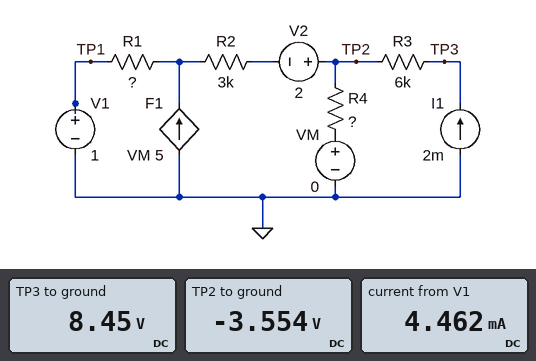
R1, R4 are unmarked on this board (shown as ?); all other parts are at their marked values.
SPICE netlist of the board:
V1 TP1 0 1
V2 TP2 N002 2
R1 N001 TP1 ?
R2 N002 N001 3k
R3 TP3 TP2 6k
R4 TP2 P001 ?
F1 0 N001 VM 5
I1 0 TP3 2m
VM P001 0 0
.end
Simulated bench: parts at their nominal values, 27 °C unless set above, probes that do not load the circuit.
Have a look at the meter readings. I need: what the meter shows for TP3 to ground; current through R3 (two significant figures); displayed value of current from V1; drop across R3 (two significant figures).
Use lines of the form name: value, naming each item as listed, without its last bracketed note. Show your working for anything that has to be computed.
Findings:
what the meter shows for TP3 to ground: 8.45 V
current through R3: (8.45 V - (-3.554 V)) / 6 kΩ = 2.0 mA
displayed value of current from V1: 4.462 mA
drop across R3: 8.45 V - (-3.554 V) = 12 V
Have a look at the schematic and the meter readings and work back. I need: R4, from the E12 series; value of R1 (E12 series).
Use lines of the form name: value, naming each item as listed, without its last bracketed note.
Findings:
R4, from the E12 series: 2.2 kΩ
value of R1: 3.9 kΩ
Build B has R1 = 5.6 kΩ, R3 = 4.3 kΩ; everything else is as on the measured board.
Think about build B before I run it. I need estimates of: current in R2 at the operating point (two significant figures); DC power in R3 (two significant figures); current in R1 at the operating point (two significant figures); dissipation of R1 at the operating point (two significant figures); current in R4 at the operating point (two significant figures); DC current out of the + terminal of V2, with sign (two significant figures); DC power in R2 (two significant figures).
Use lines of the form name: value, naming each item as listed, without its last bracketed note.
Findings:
current in R2 at the operating point: 3.2 mA
DC power in R3: 17 mW
current in R1 at the operating point: 2.7 mA
dissipation of R1 at the operating point: 41 mW
current in R4 at the operating point: 1.2 mA
DC current out of the + terminal of V2, with sign: -3.2 mA
DC power in R2: 30 mW
